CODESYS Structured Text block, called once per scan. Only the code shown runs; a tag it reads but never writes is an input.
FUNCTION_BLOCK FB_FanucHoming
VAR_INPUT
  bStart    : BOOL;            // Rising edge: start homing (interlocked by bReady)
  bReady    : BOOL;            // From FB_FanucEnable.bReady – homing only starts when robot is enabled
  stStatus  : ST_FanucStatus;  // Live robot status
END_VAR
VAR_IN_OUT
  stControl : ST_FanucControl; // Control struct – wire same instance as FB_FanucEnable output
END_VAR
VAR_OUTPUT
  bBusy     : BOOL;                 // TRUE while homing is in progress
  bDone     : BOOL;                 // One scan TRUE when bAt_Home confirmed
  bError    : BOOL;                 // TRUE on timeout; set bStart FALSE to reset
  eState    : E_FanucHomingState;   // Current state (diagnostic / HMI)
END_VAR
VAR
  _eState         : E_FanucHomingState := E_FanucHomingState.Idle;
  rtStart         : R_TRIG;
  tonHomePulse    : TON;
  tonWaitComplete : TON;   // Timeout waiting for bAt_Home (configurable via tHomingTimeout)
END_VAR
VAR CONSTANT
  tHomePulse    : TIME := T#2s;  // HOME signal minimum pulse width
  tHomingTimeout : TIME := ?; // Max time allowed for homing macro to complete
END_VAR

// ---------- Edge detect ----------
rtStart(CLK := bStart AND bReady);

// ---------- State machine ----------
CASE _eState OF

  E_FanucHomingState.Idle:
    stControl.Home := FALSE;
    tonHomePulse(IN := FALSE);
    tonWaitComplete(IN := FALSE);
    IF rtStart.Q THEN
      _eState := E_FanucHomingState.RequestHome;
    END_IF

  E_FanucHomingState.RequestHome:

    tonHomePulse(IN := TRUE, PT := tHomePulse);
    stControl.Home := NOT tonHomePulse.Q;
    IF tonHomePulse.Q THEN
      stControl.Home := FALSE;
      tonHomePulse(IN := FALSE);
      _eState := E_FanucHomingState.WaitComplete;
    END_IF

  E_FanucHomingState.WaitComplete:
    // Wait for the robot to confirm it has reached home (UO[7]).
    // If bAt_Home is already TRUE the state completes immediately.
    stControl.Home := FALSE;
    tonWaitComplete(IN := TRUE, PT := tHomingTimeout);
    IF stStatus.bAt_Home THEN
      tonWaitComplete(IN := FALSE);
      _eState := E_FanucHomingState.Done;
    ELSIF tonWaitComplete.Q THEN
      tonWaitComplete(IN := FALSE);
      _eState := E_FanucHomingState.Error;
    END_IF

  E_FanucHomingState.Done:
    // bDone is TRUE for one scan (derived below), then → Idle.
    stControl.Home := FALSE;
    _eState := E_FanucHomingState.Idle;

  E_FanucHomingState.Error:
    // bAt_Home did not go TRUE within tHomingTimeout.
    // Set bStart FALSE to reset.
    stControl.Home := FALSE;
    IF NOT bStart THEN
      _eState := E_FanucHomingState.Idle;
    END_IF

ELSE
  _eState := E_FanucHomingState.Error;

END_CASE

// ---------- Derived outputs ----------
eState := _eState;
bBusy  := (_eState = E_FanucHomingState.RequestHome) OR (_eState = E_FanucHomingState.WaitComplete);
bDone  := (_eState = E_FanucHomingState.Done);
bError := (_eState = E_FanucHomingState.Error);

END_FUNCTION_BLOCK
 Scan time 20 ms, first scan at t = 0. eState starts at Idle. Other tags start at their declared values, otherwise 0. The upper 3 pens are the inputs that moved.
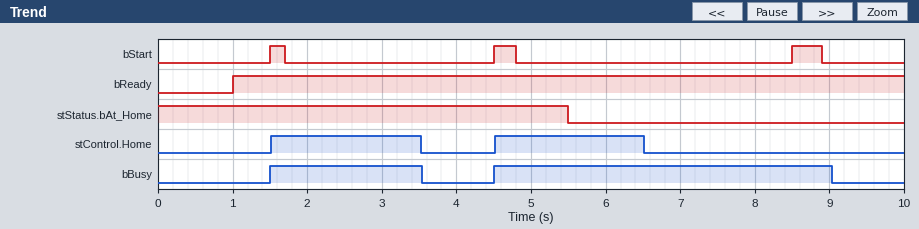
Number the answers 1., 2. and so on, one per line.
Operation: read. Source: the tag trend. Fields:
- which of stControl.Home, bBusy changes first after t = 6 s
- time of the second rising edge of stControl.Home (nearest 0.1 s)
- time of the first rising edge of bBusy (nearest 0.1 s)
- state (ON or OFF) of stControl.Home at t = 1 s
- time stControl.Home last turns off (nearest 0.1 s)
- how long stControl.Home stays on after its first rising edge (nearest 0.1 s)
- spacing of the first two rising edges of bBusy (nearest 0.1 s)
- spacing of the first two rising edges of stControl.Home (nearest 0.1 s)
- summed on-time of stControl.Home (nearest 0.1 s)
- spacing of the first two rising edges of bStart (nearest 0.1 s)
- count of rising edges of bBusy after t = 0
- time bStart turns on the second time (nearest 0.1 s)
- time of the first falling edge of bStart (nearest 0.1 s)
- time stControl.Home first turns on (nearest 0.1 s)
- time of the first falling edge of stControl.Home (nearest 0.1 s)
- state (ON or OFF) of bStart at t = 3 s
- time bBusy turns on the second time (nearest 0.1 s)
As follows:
1. stControl.Home
2. 4.5 s
3. 1.5 s
4. OFF
5. 6.5 s
6. 2.0 s
7. 3.0 s
8. 3.0 s
9. 4.0 s
10. 3.0 s
11. 2
12. 4.5 s
13. 1.7 s
14. 1.5 s
15. 3.5 s
16. OFF
17. 4.5 s
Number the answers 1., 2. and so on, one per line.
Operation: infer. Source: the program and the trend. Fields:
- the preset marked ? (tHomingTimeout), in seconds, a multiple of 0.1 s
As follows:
1. 2.5 s
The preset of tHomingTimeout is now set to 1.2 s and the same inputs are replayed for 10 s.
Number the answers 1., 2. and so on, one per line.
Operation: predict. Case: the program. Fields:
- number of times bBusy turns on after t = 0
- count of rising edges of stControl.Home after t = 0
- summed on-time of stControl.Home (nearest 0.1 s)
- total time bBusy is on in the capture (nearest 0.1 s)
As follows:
1. 3
2. 3
3. 5.5 s
4. 6.8 s
